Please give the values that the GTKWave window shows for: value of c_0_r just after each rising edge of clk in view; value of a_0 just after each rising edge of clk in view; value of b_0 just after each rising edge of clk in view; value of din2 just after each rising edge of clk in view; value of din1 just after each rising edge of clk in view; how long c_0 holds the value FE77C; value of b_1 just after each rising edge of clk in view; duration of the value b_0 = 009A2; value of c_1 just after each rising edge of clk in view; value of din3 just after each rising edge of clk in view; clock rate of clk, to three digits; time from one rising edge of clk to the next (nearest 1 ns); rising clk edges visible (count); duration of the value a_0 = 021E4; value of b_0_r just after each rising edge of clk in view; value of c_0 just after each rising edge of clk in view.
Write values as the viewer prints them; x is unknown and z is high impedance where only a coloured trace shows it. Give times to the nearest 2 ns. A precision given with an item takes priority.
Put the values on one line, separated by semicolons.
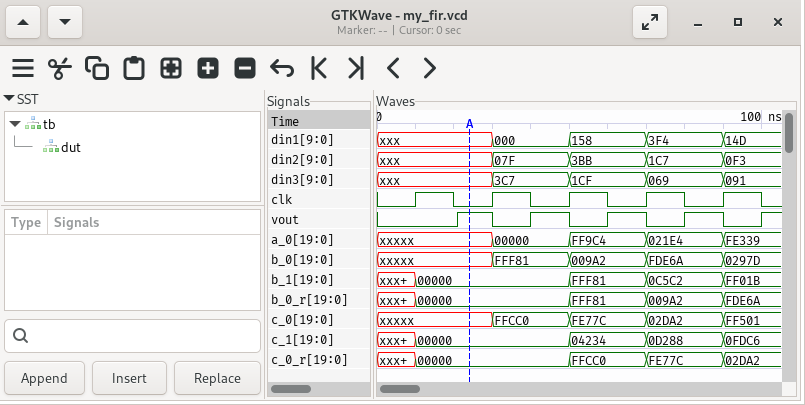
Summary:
00000, 00000, FFCC0, FE77C, 02DA2; xxxxx, 00000, FF9C4, 021E4, FE339; xxxxx, FFF81, 009A2, FDE6A, 0297D; xxx, 07F, 3BB, 1C7, 0F3; xxx, 000, 158, 3F4, 14D; 20 ns; 00000, 00000, FFF81, 0C5C2, FF01B; 20 ns; 00000, 00000, 04234, 0D288, 0FDC6; xxx, 3C7, 1CF, 069, 091; 50.0 MHz; 20 ns; 5; 20 ns; 00000, 00000, FFF81, 009A2, FDE6A; xxxxx, FFCC0, FE77C, 02DA2, FF501
